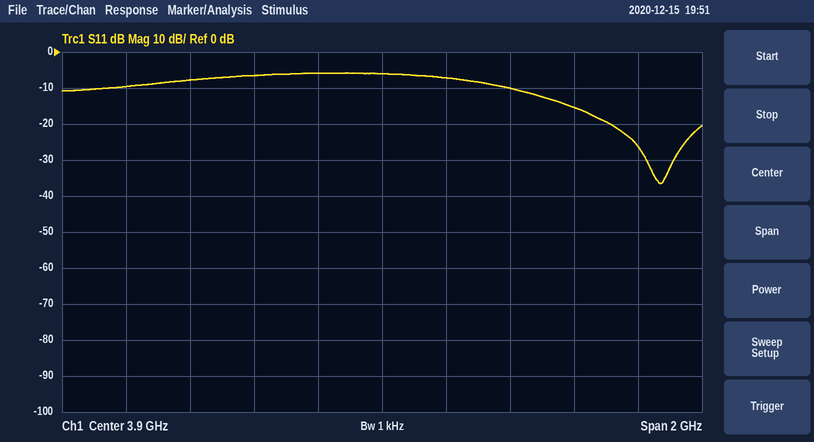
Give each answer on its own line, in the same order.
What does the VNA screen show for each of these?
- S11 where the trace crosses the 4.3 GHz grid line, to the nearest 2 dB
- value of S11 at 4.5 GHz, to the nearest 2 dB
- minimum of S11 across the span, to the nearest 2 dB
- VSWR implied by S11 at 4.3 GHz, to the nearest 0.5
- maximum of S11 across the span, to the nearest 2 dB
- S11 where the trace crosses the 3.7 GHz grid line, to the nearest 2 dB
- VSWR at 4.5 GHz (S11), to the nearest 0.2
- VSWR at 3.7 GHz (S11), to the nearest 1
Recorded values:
-10 dB
-16 dB
-36 dB
2.0
-6 dB
-6 dB
1.4
3
